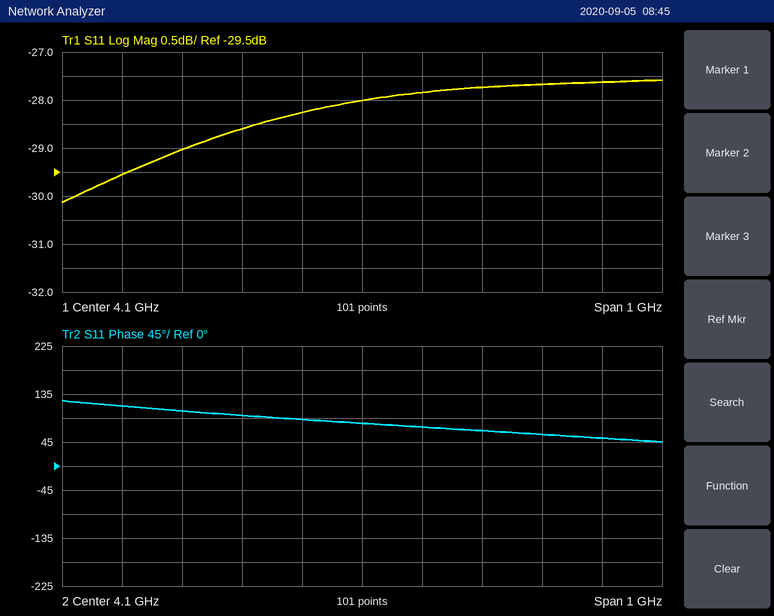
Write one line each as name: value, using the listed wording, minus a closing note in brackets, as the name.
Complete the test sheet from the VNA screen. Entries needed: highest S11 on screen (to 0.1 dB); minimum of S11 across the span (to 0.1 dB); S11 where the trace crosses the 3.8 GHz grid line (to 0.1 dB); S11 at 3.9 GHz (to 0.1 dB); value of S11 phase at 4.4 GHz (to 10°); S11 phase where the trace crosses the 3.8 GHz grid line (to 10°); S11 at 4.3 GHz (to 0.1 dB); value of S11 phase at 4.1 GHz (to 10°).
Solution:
highest S11 on screen: -27.6 dB
minimum of S11 across the span: -30.1 dB
S11 where the trace crosses the 3.8 GHz grid line: -29.0 dB
S11 at 3.9 GHz: -28.6 dB
value of S11 phase at 4.4 GHz: 60°
S11 phase where the trace crosses the 3.8 GHz grid line: 100°
S11 at 4.3 GHz: -27.7 dB
value of S11 phase at 4.1 GHz: 80°
